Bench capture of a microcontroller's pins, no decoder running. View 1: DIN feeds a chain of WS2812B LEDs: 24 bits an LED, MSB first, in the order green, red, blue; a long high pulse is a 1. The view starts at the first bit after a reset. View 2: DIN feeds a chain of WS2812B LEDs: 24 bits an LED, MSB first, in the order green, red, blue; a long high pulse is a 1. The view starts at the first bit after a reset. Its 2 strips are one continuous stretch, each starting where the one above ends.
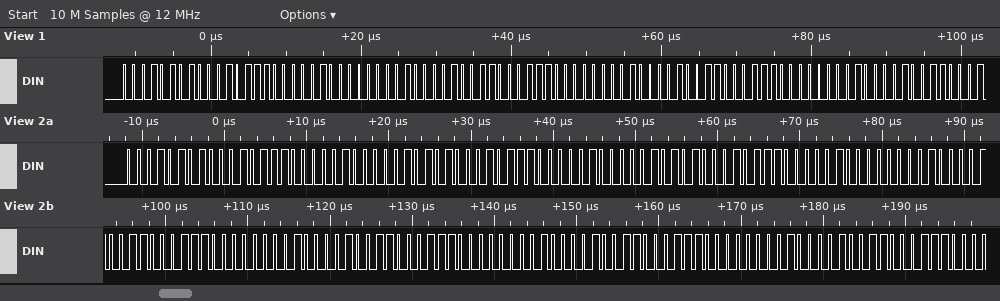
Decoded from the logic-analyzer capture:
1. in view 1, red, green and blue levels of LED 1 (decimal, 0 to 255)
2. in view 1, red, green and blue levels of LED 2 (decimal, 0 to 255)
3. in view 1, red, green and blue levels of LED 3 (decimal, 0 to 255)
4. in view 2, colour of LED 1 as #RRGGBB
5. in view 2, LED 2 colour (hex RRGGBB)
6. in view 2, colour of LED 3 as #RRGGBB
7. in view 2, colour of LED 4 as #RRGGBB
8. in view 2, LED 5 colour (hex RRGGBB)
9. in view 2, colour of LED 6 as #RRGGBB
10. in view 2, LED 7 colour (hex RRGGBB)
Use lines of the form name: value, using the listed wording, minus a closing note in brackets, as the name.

in view 1, red, green and blue levels of LED 1: 23, 21, 4
in view 1, red, green and blue levels of LED 2: 19, 2, 28
in view 1, red, green and blue levels of LED 3: 19, 2, 28
in view 2, colour of LED 1 as #RRGGBB: #171504
in view 2, LED 2 colour: #171504
in view 2, colour of LED 3 as #RRGGBB: #171504
in view 2, colour of LED 4 as #RRGGBB: #13021C
in view 2, LED 5 colour: #13021C
in view 2, colour of LED 6 as #RRGGBB: #13021C
in view 2, LED 7 colour: #13021C
